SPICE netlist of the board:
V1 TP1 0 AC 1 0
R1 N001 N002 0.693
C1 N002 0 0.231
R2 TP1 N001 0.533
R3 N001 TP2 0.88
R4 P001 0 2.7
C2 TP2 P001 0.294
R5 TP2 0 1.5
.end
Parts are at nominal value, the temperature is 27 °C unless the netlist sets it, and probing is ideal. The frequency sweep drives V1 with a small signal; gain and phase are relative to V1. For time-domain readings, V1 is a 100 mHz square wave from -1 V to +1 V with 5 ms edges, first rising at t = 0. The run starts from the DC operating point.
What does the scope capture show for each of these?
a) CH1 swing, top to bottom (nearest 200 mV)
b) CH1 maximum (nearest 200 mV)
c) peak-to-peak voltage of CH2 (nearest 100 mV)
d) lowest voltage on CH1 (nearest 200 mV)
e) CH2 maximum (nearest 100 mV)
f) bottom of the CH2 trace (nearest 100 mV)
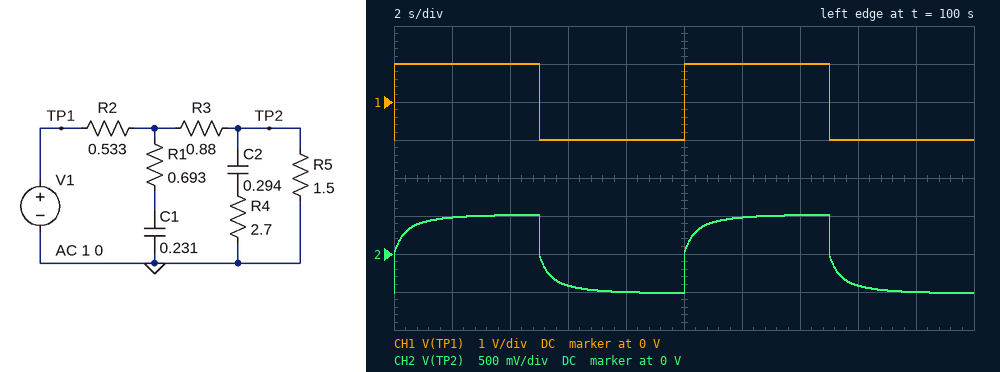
2.0 V
1.0 V
1.0 V
-1.0 V
500 mV
-500 mV
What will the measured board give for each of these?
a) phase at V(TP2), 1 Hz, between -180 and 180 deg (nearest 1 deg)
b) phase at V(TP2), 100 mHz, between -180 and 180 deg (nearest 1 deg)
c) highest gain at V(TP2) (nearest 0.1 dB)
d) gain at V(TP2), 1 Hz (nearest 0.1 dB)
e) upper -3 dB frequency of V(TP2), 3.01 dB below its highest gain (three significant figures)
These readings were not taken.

-15 deg
-9 deg
-5.8 dB
-10.3 dB
490 mHz
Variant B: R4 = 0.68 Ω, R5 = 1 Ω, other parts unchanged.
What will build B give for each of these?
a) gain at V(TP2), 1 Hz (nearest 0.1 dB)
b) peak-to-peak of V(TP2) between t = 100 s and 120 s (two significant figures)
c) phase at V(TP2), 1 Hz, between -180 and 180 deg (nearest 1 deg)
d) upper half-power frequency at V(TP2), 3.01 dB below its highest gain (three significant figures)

-14.0 dB
830 mV
-27 deg
443 mHz
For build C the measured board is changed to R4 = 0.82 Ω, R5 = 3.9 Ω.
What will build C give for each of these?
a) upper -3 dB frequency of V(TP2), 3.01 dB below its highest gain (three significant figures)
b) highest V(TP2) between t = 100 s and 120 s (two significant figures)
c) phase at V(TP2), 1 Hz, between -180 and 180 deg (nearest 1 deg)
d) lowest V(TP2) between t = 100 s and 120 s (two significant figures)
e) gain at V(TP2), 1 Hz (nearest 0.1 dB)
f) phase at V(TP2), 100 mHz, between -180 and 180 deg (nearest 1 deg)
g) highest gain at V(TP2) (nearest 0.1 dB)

300 mHz
730 mV
-29 deg
-730 mV
-11.1 dB
-14 deg
-2.7 dB
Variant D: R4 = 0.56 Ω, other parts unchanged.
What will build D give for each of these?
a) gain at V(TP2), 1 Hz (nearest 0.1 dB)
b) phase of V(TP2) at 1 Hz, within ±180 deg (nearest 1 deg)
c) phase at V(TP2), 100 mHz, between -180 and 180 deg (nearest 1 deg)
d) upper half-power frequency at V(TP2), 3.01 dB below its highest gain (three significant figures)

-13.3 dB
-33 deg
-11 deg
396 mHz
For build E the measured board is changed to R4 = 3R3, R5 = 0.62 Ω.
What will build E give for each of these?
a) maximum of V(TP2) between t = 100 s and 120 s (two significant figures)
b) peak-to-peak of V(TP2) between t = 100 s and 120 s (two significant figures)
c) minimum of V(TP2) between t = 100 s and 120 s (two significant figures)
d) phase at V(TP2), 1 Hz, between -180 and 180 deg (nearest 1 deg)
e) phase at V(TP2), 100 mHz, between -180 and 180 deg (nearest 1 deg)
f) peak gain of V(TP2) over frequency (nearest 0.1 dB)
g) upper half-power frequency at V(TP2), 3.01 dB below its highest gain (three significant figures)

300 mV
610 mV
-300 mV
-13 deg
-6 deg
-10.3 dB
819 mHz
